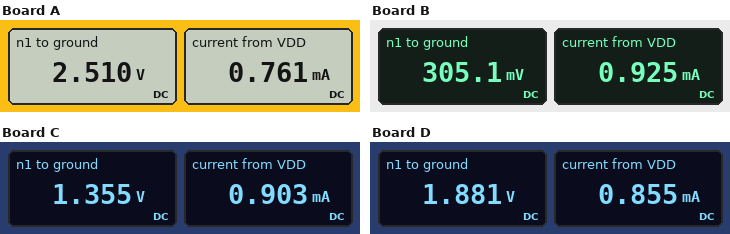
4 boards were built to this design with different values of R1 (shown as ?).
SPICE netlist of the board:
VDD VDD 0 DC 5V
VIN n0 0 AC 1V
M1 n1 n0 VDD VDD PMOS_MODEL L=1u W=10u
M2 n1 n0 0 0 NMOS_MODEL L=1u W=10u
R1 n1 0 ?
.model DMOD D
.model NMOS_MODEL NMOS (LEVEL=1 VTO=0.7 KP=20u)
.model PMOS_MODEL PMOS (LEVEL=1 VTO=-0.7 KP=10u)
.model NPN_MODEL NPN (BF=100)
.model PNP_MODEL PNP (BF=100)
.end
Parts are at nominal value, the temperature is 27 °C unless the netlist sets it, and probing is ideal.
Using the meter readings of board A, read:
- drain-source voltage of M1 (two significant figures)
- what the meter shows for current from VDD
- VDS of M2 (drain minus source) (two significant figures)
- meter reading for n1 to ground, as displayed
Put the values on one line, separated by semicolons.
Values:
-2.5 V; 0.761 mA; 2.5 V; 2.510 V
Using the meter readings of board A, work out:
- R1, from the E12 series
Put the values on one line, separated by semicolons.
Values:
3.3 kΩ
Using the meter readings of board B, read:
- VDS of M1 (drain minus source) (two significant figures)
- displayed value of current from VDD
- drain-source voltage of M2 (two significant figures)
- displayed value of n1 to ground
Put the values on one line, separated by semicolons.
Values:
-4.7 V; 0.925 mA; 310 mV; 305.1 mV
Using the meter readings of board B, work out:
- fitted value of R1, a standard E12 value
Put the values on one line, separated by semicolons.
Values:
330 Ω
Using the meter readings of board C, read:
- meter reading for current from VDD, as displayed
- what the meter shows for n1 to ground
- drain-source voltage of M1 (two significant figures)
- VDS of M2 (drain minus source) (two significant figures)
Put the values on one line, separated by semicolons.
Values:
0.903 mA; 1.355 V; -3.6 V; 1.4 V
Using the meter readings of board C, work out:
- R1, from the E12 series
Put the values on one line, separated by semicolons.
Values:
1.5 kΩ
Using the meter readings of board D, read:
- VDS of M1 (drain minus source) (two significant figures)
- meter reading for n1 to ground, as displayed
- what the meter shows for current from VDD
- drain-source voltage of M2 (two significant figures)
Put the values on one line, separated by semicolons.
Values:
-3.1 V; 1.881 V; 0.855 mA; 1.9 V
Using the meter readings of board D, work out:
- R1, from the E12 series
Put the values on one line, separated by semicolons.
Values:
2.2 kΩ
